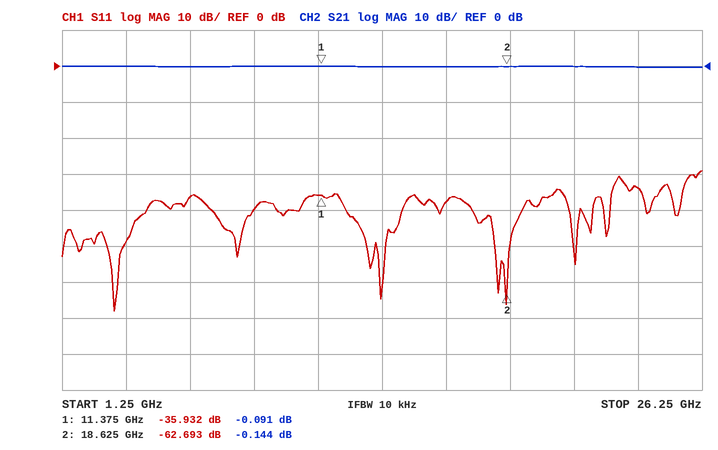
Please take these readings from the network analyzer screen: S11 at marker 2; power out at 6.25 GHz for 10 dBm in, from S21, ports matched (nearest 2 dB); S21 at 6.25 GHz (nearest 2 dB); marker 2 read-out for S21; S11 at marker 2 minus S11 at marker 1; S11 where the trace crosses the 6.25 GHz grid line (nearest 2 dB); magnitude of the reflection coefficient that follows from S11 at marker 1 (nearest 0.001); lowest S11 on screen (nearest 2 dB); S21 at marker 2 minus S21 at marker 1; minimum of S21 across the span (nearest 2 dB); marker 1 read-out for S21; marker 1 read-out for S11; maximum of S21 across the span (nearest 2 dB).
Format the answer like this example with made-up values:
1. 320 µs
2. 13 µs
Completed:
1. -62.693 dB
2. 10 dBm
3. 0 dB
4. -0.144 dB
5. -26.761 dB
6. -36 dB
7. 0.016
8. -68 dB
9. -0.053 dB
10. 0 dB
11. -0.091 dB
12. -35.932 dB
13. 0 dB
